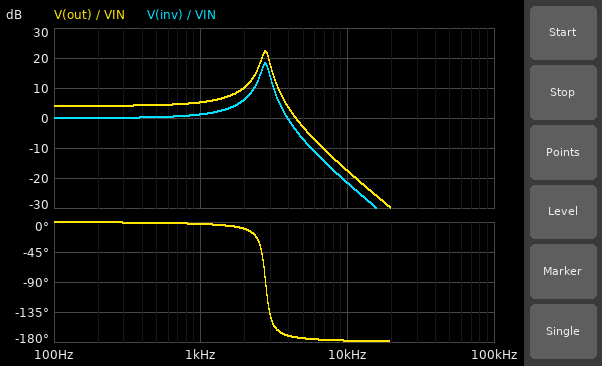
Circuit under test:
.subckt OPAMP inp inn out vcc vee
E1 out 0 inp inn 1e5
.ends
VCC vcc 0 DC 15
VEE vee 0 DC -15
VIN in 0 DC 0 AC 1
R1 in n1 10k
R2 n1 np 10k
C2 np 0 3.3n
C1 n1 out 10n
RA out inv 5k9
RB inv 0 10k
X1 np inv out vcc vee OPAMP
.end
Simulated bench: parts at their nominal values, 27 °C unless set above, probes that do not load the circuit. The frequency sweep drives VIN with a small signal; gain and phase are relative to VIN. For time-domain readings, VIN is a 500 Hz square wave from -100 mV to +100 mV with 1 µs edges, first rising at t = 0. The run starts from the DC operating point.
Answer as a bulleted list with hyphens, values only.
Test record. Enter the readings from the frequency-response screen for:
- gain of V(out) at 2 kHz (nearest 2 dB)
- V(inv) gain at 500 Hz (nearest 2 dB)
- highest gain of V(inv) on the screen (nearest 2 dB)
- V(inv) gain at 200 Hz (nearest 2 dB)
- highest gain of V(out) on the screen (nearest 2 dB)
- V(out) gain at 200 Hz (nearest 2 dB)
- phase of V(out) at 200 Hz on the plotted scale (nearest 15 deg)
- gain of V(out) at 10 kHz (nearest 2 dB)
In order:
- 10 dB
- 0 dB
- 18 dB
- 0 dB
- 22 dB
- 4 dB
- 0 deg
- -18 dB
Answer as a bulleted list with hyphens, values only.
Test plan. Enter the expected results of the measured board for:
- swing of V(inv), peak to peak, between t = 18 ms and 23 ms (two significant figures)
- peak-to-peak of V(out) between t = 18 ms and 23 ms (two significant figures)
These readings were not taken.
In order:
- 510 mV
- 810 mV
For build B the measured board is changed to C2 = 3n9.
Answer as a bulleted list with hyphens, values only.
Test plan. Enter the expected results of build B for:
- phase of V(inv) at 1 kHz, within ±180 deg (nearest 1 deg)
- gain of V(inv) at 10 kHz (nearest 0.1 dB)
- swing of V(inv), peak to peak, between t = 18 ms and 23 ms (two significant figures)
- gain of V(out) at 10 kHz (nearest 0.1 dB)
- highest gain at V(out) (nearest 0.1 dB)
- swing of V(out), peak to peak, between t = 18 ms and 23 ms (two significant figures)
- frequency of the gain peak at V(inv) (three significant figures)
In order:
- -8 deg
- -23.2 dB
- 470 mV
- -19.2 dB
- 14.5 dB
- 750 mV
- 2.49 kHz
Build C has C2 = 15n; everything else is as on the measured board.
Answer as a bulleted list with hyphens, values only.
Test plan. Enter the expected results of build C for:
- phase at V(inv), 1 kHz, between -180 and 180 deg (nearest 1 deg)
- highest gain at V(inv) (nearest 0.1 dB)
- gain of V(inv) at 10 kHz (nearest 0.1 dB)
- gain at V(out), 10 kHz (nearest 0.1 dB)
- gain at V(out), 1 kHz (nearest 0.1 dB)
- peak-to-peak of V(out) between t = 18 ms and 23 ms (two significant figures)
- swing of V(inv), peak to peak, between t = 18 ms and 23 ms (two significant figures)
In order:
- -75 deg
- 0 dB
- -35.6 dB
- -31.6 dB
- 0.1 dB
- 320 mV
- 200 mV
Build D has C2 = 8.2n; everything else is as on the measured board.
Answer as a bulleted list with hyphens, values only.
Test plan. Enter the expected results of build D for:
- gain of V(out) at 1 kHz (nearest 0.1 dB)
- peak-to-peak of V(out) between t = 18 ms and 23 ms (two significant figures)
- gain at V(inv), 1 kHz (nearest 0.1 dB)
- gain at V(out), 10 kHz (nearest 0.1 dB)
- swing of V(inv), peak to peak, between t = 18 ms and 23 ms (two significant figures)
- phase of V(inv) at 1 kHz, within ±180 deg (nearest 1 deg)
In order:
- 4.5 dB
- 390 mV
- 0.5 dB
- -26.1 dB
- 240 mV
- -44 deg
